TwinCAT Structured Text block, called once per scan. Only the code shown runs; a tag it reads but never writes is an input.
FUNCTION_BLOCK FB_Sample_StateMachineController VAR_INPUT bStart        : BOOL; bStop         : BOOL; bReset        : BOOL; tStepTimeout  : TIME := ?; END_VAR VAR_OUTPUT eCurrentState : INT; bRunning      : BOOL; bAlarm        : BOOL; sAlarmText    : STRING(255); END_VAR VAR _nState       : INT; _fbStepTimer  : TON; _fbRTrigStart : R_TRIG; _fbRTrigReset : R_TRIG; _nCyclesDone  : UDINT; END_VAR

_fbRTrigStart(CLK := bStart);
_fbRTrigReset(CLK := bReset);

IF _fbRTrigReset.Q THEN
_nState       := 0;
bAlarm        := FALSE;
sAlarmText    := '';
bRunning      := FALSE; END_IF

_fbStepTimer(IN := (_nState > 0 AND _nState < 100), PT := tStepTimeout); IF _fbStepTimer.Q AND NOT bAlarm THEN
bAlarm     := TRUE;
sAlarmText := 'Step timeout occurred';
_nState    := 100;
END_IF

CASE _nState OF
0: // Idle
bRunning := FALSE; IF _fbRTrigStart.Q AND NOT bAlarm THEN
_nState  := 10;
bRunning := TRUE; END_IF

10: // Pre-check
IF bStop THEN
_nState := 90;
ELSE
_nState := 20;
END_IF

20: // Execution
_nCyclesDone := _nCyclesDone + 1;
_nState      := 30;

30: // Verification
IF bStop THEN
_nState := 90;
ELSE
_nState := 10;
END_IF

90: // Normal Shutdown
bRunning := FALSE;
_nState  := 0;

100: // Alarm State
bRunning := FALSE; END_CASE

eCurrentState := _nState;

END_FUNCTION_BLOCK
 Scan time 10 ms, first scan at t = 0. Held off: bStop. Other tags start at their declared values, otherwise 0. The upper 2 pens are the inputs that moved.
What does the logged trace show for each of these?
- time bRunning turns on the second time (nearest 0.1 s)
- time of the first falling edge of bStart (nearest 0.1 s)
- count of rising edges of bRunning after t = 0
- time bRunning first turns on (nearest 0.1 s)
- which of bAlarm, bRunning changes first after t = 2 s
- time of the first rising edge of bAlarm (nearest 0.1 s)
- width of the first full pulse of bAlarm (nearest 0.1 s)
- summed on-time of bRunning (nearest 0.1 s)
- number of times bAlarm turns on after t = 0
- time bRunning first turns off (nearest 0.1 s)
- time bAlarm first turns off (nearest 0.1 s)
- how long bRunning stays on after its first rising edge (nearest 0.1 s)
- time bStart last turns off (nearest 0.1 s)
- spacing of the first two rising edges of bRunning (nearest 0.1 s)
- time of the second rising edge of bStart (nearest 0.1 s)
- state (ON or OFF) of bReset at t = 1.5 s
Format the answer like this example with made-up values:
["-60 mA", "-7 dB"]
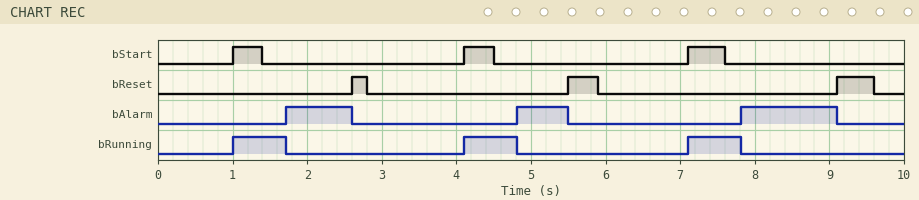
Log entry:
["4.1 s", "1.4 s", "3", "1.0 s", "bAlarm", "1.7 s", "0.9 s", "2.1 s", "3", "1.7 s", "2.6 s", "0.7 s", "7.6 s", "3.1 s", "4.1 s", "OFF"]
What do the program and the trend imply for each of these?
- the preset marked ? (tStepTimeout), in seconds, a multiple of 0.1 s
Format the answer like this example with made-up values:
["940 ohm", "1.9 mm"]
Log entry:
["0.7 s"]
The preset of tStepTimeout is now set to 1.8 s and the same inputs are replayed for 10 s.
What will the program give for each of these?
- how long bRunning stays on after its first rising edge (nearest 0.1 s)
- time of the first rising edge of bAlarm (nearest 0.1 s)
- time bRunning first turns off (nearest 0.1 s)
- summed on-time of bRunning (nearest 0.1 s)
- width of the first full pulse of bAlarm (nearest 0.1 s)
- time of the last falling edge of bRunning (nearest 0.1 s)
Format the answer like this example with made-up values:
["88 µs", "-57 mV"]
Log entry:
["1.6 s", "8.9 s", "2.6 s", "4.8 s", "0.2 s", "8.9 s"]
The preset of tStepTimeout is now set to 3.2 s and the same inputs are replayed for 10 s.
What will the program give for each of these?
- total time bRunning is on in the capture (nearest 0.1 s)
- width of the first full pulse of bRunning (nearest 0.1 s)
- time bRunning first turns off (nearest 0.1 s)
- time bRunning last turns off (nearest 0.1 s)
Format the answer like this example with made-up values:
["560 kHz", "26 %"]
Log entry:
["5.0 s", "1.6 s", "2.6 s", "9.1 s"]
